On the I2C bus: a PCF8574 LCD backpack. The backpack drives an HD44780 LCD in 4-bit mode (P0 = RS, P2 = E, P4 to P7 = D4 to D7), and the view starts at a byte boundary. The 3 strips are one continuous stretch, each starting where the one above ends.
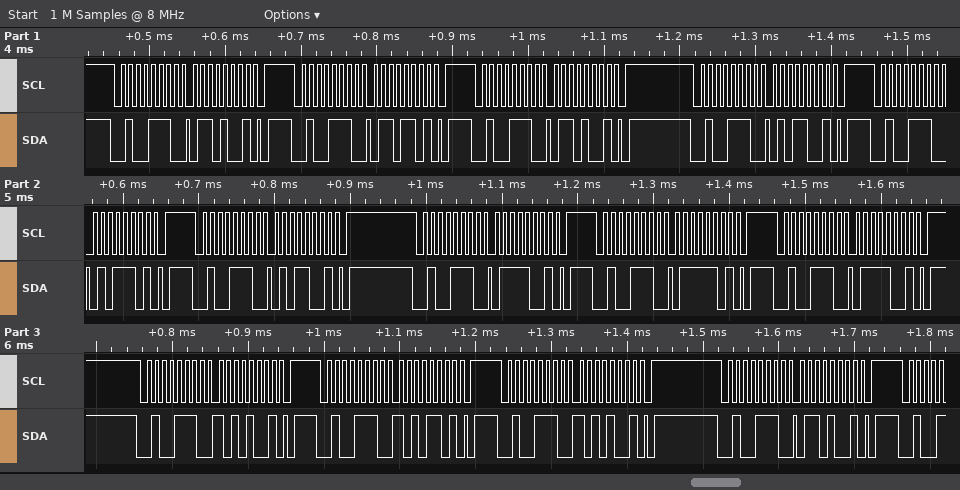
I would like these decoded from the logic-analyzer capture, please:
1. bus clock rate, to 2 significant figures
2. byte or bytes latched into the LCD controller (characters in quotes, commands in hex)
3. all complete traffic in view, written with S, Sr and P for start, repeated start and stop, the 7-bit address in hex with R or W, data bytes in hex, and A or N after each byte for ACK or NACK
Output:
100 kHz
'e' 'z'
S 27W A 69 A P S 27W A 6D A P S 27W A 69 A P S 27W A 59 A P S 27W A 5D A P S 27W A 59 A P S 27W A 79 A P S 27W A 7D A P S 27W A 79 A P S 27W A A9 A P S 27W A AD A P S 27W A A9 A P S 27W A 69 A P
